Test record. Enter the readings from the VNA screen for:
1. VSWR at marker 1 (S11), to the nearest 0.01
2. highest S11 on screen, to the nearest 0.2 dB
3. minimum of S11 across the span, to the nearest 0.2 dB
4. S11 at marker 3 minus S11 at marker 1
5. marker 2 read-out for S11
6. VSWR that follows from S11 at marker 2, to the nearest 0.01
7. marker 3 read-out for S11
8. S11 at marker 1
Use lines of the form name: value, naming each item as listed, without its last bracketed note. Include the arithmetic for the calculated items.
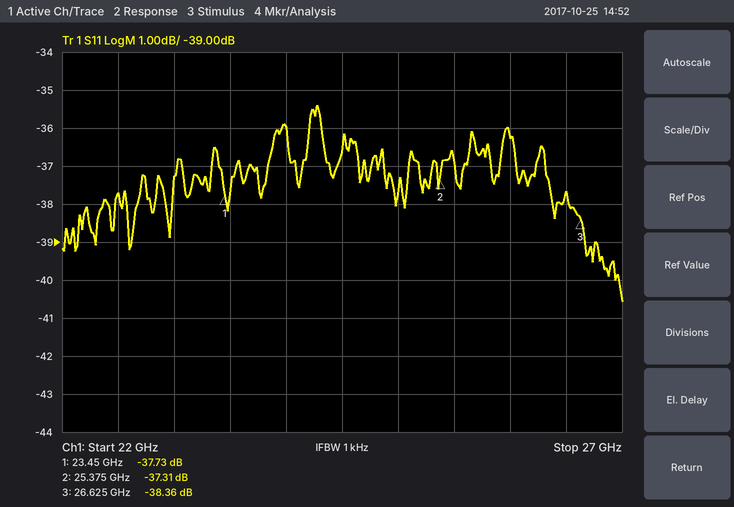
VSWR at marker 1 (S11), to the nearest 0.01: (1 + 0.0130)/(1 − 0.0130) ≈ 1.03
highest S11 on screen, to the nearest 0.2 dB: -35.4 dB
minimum of S11 across the span, to the nearest 0.2 dB: -40.6 dB
S11 at marker 3 minus S11 at marker 1: -38.36 − (-37.73) = -0.63 dB
marker 2 read-out for S11: -37.31 dB
VSWR that follows from S11 at marker 2, to the nearest 0.01: (1 + 0.0136)/(1 − 0.0136) ≈ 1.03
marker 3 read-out for S11: -38.36 dB
S11 at marker 1: -37.73 dB
